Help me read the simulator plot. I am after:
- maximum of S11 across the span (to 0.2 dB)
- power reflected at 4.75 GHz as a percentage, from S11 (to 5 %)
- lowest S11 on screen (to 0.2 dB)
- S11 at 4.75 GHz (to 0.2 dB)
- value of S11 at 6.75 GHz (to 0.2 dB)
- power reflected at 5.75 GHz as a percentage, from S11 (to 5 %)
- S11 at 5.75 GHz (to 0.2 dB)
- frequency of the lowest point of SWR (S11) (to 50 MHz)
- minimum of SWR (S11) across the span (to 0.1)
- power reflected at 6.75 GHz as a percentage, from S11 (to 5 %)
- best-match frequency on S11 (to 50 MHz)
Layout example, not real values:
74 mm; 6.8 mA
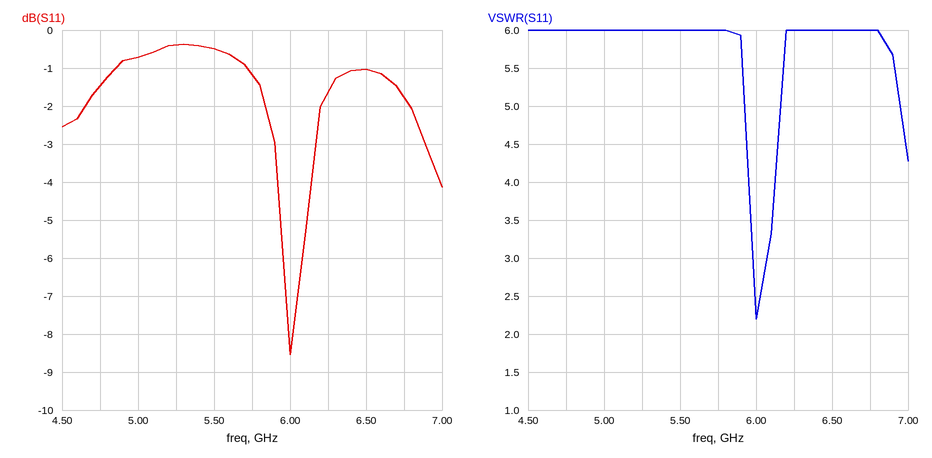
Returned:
-0.4 dB; 70 %; -8.6 dB; -1.4 dB; -1.8 dB; 75 %; -1.2 dB; 6.00 GHz; 2.2; 65 %; 6.00 GHz
